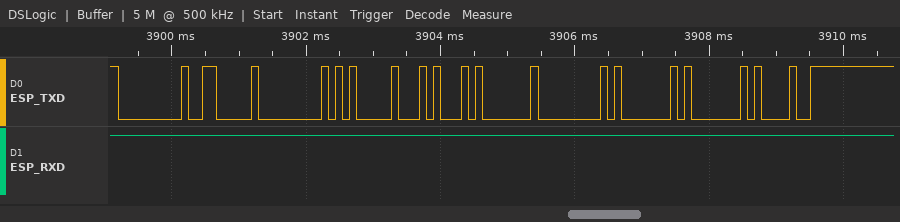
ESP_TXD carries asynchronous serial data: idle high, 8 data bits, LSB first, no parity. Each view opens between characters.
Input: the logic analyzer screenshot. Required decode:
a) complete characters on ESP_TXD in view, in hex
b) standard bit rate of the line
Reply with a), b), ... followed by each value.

a) 00, 06, 00, 05, 14, 01, 00, 01, 01, 21
b) 9600 baud
